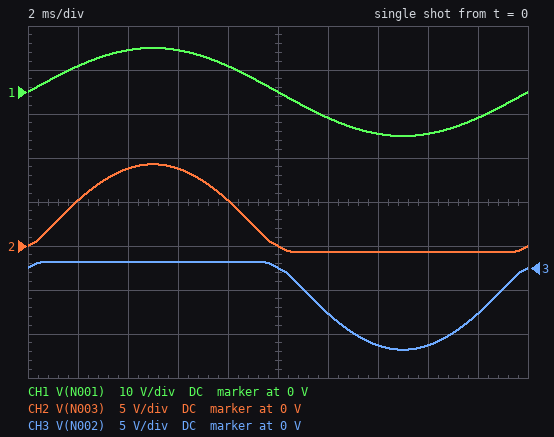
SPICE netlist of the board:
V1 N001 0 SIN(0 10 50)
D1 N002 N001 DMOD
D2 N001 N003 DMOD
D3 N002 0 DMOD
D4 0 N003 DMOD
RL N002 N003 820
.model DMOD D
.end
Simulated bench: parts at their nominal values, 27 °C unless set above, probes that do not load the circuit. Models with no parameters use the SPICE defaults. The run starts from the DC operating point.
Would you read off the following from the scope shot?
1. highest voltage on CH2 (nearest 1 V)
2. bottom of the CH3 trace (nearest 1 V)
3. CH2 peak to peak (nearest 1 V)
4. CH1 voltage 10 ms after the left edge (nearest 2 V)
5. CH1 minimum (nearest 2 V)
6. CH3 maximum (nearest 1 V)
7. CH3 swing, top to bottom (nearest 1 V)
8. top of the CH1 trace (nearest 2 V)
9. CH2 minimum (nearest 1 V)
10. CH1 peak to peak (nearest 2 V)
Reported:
9 V
-9 V
10 V
0 V
-10 V
1 V
10 V
10 V
-1 V
20 V
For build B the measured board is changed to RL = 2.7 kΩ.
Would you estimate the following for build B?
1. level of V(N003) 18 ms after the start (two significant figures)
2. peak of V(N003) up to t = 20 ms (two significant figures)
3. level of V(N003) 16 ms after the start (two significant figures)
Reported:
-670 mV
9.3 V
-680 mV
